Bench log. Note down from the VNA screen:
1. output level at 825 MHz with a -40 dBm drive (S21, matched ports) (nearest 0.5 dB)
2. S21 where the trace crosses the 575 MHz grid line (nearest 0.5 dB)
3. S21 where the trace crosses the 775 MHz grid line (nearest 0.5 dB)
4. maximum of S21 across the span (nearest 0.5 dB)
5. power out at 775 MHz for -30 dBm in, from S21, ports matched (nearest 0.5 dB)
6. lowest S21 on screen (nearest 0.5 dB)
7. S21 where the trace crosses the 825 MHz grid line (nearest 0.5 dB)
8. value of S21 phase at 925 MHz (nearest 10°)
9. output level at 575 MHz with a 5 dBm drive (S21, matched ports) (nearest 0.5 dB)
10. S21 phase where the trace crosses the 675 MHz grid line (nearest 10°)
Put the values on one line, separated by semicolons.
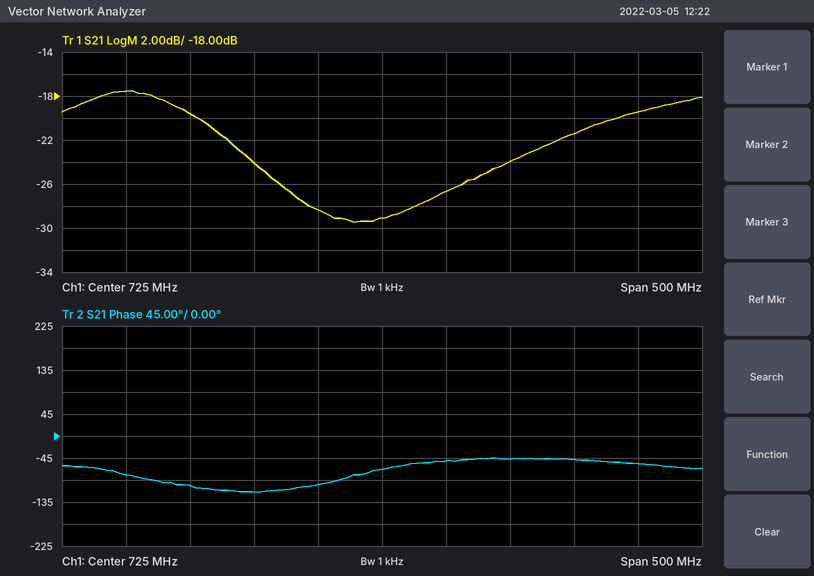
-64.0 dBm; -19.5 dB; -26.5 dB; -17.5 dB; -56.5 dBm; -29.5 dB; -24.0 dB; -60°; -14.5 dBm; -100°
